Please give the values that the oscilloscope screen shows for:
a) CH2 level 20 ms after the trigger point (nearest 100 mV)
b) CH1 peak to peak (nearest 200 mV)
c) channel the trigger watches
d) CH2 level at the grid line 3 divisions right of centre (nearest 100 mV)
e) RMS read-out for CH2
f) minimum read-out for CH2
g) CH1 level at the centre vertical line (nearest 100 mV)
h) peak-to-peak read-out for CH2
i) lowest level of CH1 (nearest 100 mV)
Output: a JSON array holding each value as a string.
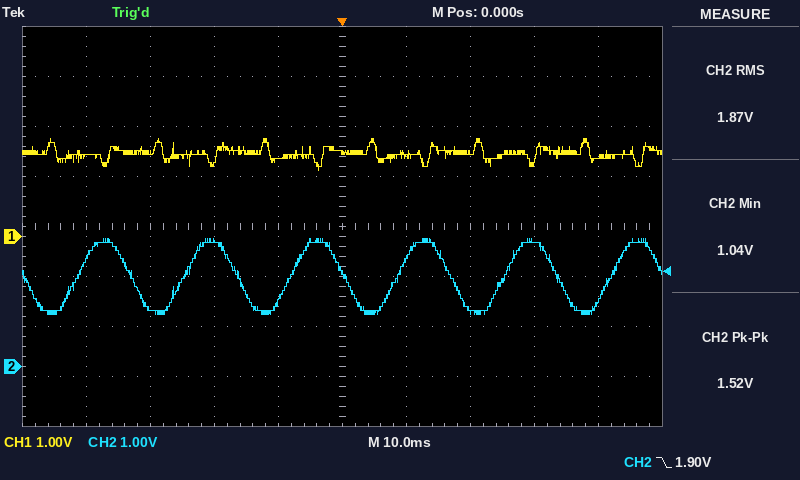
["1.1 V", "600 mV", "CH2", "2.5 V", "1.87 V", "1.04 V", "1.7 V", "1.52 V", "1.3 V"]
